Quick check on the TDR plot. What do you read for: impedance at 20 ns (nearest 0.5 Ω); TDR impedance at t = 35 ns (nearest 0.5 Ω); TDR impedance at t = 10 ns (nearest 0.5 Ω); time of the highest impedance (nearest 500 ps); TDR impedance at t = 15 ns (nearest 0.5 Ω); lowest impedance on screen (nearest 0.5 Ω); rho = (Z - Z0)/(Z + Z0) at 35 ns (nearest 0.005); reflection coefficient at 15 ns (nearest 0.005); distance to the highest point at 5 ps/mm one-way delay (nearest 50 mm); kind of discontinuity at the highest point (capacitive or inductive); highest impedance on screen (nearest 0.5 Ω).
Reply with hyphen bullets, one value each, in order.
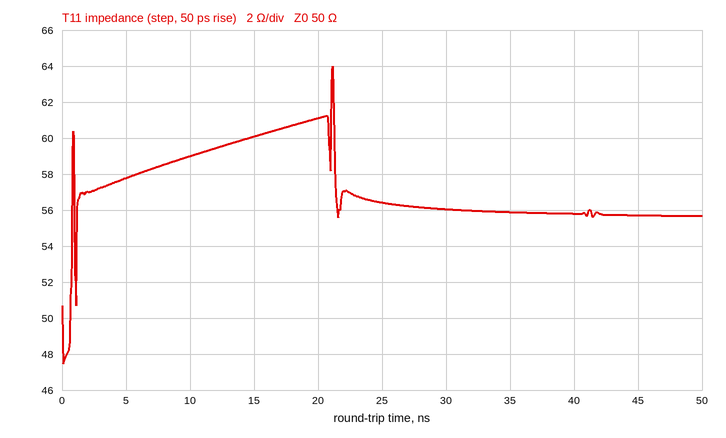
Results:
- 61.0 Ω
- 56.0 Ω
- 59.0 Ω
- 21.0 ns
- 60.0 Ω
- 47.5 Ω
- +0.055
- +0.090
- 2.10 m
- inductive
- 64.0 Ω
